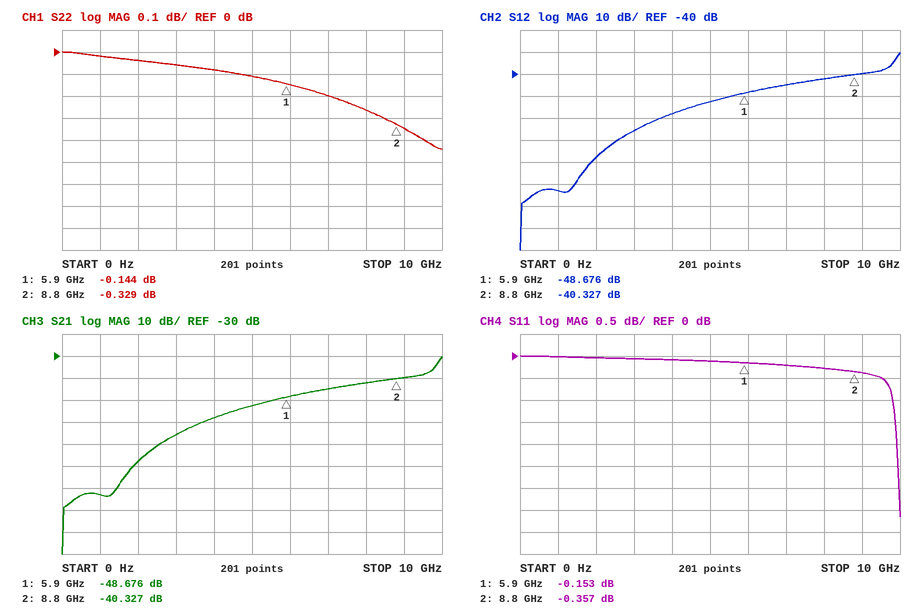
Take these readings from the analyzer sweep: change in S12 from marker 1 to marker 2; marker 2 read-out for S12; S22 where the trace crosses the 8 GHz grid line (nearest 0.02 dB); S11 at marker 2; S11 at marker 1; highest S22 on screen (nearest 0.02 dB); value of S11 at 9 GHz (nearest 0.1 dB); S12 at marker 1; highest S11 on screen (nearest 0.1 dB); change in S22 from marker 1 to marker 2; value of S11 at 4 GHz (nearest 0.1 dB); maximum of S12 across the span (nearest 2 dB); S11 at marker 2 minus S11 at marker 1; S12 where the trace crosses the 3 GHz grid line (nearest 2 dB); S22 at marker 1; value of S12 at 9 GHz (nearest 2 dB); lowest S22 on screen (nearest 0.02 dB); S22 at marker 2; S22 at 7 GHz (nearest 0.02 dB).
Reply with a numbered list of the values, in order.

1. 8.349 dB
2. -40.327 dB
3. -0.26 dB
4. -0.357 dB
5. -0.153 dB
6. 0.00 dB
7. -0.4 dB
8. -48.676 dB
9. 0.0 dB
10. -0.185 dB
11. -0.1 dB
12. -30 dB
13. -0.204 dB
14. -66 dB
15. -0.144 dB
16. -40 dB
17. -0.44 dB
18. -0.329 dB
19. -0.20 dB
